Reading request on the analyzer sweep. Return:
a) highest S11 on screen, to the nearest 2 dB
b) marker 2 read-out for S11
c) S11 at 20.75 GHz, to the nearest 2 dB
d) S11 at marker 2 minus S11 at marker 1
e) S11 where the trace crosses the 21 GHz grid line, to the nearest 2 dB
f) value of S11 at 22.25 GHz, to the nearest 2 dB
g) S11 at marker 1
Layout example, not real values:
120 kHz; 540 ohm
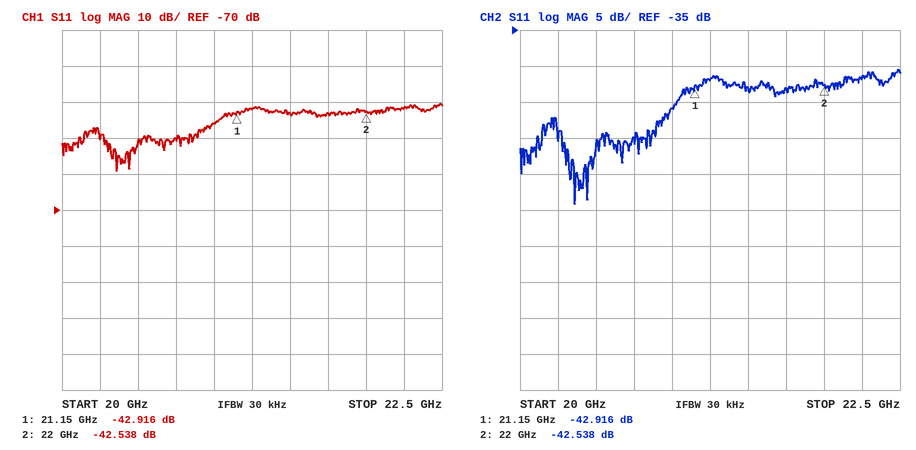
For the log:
-40 dB; -42.538 dB; -50 dB; 0.378 dB; -46 dB; -42 dB; -42.916 dB
